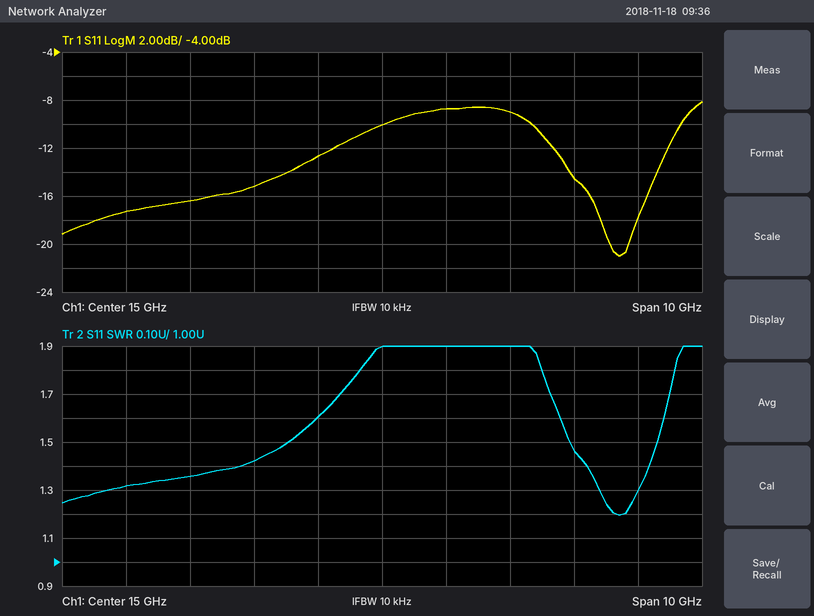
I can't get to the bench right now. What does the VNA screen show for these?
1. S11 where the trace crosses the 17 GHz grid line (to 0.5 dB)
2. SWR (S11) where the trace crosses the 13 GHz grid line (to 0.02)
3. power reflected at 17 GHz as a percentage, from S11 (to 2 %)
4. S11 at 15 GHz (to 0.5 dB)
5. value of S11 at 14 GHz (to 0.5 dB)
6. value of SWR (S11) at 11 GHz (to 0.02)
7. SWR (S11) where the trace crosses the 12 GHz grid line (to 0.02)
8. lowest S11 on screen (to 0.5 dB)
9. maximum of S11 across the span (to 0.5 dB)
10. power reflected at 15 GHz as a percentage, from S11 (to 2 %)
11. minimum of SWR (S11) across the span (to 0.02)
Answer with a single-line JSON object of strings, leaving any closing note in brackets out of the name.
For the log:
{"S11 where the trace crosses the 17 GHz grid line": "-9.0 dB", "SWR (S11) where the trace crosses the 13 GHz grid line": "1.42", "power reflected at 17 GHz as a percentage, from S11": "12 %", "S11 at 15 GHz": "-10.0 dB", "value of S11 at 14 GHz": "-12.5 dB", "value of SWR (S11) at 11 GHz": "1.32", "SWR (S11) where the trace crosses the 12 GHz grid line": "1.36", "lowest S11 on screen": "-21.0 dB", "maximum of S11 across the span": "-8.0 dB", "power reflected at 15 GHz as a percentage, from S11": "10 %", "minimum of SWR (S11) across the span": "1.20"}
